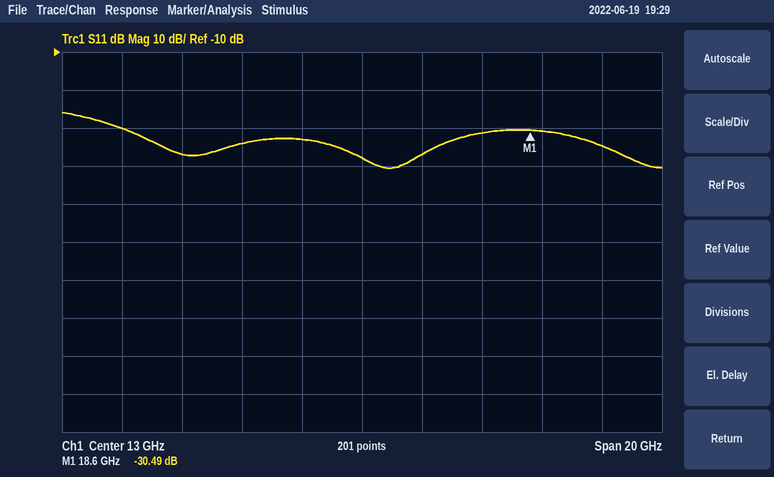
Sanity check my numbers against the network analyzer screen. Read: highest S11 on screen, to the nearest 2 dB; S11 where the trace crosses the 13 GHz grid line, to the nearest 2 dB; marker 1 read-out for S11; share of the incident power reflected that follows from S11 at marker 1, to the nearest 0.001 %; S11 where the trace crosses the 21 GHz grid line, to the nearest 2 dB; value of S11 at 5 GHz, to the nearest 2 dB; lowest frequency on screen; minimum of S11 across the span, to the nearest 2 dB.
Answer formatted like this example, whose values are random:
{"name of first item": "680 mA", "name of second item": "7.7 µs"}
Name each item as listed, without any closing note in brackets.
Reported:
{"highest S11 on screen, to the nearest 2 dB": "-26 dB", "S11 where the trace crosses the 13 GHz grid line, to the nearest 2 dB": "-38 dB", "marker 1 read-out for S11": "-30.49 dB", "share of the incident power reflected that follows from S11 at marker 1, to the nearest 0.001 %": "0.089 %", "S11 where the trace crosses the 21 GHz grid line, to the nearest 2 dB": "-34 dB", "value of S11 at 5 GHz, to the nearest 2 dB": "-30 dB", "lowest frequency on screen": "3 GHz", "minimum of S11 across the span, to the nearest 2 dB": "-40 dB"}
